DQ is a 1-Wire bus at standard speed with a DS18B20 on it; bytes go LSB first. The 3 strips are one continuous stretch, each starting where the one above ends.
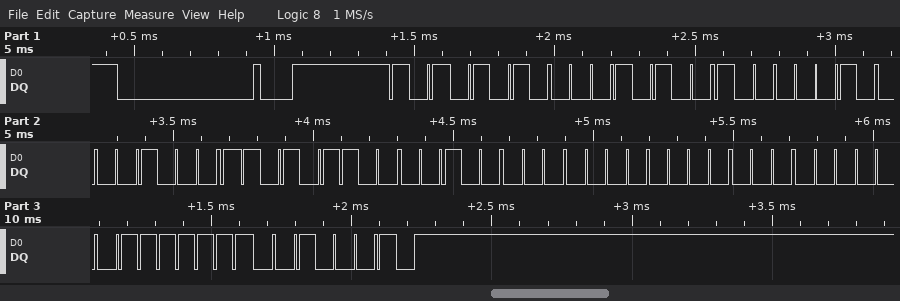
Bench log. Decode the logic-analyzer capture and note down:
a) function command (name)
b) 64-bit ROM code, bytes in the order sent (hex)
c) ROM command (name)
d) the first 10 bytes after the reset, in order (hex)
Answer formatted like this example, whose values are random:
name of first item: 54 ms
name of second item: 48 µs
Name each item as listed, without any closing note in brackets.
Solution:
function command: Convert T
64-bit ROM code, bytes in the order sent: 28 41 88 35 04 00 00 FE
ROM command: Match ROM
the first 10 bytes after the reset, in order: 55 28 41 88 35 04 00 00 FE 44
